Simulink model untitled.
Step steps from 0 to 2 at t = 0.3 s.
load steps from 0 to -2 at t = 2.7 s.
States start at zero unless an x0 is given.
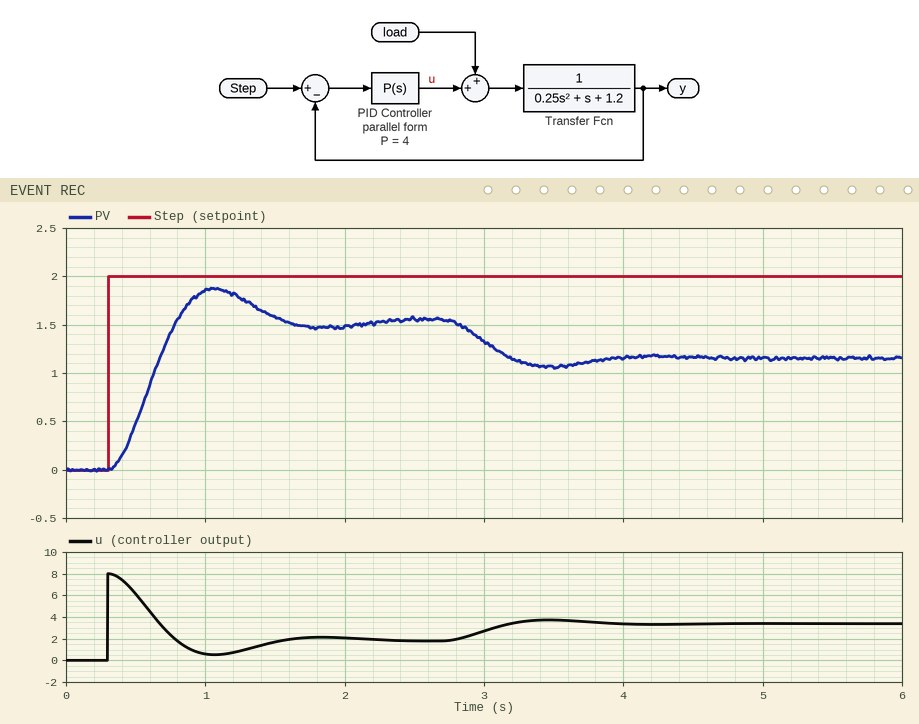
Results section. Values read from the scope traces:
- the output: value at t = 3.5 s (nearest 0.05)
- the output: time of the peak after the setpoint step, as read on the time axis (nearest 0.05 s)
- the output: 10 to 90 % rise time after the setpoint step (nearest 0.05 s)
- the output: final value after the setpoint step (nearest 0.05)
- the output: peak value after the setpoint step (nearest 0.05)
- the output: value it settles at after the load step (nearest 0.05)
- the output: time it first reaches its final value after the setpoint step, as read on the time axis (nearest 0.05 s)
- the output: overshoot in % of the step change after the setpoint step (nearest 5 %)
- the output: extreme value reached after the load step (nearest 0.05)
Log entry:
1.05
1.05 s
0.35 s
1.55
1.85
1.15
0.80 s
20 %
1.05
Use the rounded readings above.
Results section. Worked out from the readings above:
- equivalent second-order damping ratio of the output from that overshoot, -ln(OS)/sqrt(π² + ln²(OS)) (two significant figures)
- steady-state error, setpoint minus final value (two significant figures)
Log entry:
0.46
0.45
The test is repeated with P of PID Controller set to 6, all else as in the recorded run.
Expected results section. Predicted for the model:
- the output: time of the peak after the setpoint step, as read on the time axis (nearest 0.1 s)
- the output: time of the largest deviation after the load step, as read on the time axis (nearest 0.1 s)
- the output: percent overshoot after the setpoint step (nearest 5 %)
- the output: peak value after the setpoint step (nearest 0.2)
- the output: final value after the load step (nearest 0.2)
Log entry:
0.9 s
3.3 s
30 %
2.2
1.4
